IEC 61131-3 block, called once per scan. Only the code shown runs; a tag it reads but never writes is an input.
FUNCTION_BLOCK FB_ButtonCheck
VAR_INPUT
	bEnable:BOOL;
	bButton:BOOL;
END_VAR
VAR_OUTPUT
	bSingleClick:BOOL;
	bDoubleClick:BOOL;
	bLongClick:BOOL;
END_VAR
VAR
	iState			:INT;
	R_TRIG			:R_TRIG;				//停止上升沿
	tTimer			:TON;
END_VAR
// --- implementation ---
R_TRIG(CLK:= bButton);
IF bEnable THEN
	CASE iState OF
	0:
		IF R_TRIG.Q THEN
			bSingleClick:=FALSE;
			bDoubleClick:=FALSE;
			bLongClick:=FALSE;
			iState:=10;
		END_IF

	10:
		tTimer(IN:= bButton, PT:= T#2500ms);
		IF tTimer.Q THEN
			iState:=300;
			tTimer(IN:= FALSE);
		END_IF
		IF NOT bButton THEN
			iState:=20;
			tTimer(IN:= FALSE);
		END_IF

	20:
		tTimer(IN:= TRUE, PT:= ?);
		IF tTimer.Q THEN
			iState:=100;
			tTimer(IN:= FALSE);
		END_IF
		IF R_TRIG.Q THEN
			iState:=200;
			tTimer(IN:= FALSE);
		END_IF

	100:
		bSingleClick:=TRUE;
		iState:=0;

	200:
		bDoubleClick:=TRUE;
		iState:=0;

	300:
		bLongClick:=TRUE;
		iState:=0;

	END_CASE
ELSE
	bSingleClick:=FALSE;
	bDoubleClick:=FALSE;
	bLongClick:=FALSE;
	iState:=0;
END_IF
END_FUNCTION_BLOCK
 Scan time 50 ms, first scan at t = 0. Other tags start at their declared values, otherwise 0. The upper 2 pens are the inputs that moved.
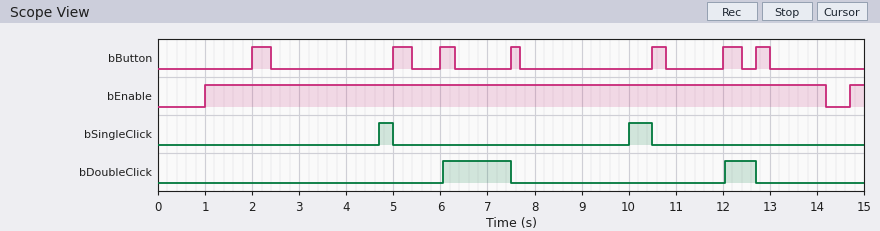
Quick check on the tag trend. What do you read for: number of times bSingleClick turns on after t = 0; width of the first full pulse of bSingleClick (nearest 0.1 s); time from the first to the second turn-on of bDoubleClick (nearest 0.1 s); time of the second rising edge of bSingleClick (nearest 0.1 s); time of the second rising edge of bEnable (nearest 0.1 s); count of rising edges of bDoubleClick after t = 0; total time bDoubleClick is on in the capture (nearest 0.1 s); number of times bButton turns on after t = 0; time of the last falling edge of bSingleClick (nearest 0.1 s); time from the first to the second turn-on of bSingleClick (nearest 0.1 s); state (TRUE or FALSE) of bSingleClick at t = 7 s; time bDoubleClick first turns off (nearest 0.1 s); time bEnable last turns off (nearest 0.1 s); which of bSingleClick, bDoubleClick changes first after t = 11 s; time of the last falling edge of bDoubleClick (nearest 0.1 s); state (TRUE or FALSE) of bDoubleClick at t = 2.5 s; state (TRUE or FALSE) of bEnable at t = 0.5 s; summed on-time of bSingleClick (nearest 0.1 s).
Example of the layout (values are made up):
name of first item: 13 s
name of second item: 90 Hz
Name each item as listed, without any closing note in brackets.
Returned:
number of times bSingleClick turns on after t = 0: 2
width of the first full pulse of bSingleClick: 0.3 s
time from the first to the second turn-on of bDoubleClick: 6.0 s
time of the second rising edge of bSingleClick: 10.0 s
time of the second rising edge of bEnable: 14.7 s
count of rising edges of bDoubleClick after t = 0: 2
total time bDoubleClick is on in the capture: 2.1 s
number of times bButton turns on after t = 0: 7
time of the last falling edge of bSingleClick: 10.5 s
time from the first to the second turn-on of bSingleClick: 5.3 s
state (TRUE or FALSE) of bSingleClick at t = 7 s: FALSE
time bDoubleClick first turns off: 7.5 s
time bEnable last turns off: 14.2 s
which of bSingleClick, bDoubleClick changes first after t = 11 s: bDoubleClick
time of the last falling edge of bDoubleClick: 12.7 s
state (TRUE or FALSE) of bDoubleClick at t = 2.5 s: FALSE
state (TRUE or FALSE) of bEnable at t = 0.5 s: FALSE
summed on-time of bSingleClick: 0.8 s
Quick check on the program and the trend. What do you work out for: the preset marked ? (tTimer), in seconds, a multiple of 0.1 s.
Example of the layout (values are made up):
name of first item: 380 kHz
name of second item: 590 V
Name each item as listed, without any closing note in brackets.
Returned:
the preset marked ? (tTimer), in seconds, a multiple of 0.1 s: 2.2 s
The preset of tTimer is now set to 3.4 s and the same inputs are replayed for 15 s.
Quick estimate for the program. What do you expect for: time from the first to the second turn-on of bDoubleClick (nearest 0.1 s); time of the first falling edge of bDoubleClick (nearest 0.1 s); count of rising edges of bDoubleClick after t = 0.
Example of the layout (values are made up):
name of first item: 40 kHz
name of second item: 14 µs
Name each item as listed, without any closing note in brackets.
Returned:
time from the first to the second turn-on of bDoubleClick: 2.5 s
time of the first falling edge of bDoubleClick: 6.0 s
count of rising edges of bDoubleClick after t = 0: 3
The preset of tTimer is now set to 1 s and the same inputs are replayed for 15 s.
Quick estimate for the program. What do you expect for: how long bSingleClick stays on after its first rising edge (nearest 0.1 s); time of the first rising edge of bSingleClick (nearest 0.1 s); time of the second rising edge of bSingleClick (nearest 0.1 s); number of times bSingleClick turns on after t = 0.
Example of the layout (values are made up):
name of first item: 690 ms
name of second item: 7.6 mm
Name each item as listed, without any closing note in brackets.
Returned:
how long bSingleClick stays on after its first rising edge: 1.5 s
time of the first rising edge of bSingleClick: 3.5 s
time of the second rising edge of bSingleClick: 8.8 s
number of times bSingleClick turns on after t = 0: 3
